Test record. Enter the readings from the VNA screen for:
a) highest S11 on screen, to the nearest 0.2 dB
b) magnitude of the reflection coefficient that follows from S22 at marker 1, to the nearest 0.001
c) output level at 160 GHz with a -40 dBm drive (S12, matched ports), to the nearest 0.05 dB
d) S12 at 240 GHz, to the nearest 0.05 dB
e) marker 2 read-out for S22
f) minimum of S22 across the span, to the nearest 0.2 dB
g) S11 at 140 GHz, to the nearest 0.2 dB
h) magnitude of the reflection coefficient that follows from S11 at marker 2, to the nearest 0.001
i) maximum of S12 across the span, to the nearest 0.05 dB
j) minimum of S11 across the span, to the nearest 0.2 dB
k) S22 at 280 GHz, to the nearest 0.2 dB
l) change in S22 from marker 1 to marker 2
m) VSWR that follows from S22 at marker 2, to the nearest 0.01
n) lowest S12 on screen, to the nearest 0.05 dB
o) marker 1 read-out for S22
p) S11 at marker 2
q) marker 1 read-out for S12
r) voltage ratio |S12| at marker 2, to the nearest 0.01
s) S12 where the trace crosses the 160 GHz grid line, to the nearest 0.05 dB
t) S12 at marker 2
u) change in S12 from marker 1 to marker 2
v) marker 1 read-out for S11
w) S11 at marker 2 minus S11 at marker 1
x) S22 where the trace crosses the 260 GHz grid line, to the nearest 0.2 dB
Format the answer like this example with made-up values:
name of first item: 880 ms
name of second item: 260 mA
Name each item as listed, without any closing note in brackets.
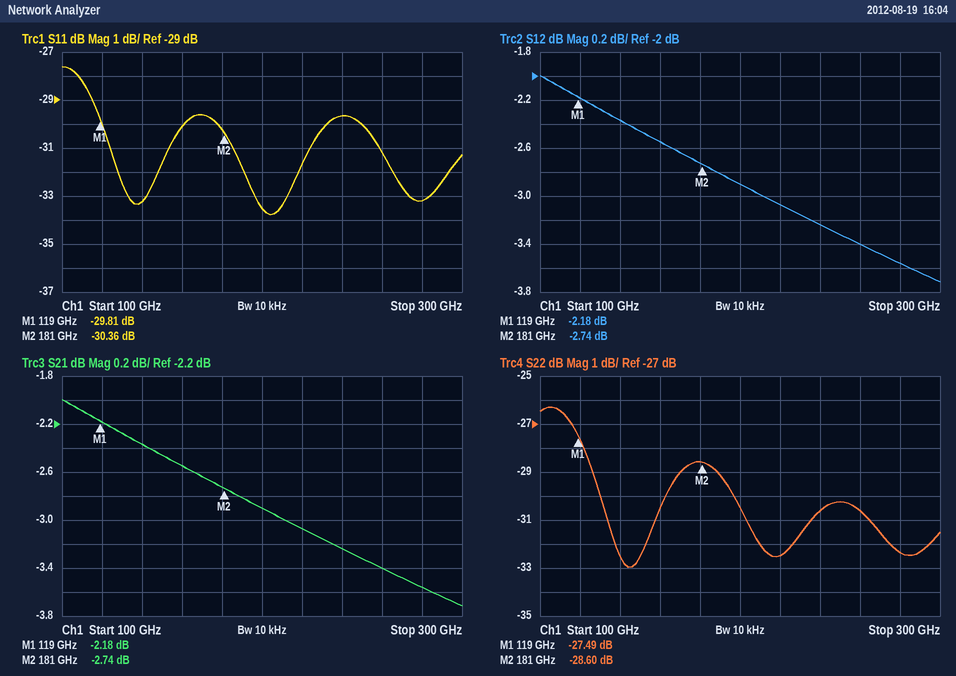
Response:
highest S11 on screen, to the nearest 0.2 dB: -27.6 dB
magnitude of the reflection coefficient that follows from S22 at marker 1, to the nearest 0.001: 0.042
output level at 160 GHz with a -40 dBm drive (S12, matched ports), to the nearest 0.05 dB: -42.55 dBm
S12 at 240 GHz, to the nearest 0.05 dB: -3.25 dB
marker 2 read-out for S22: -28.60 dB
minimum of S22 across the span, to the nearest 0.2 dB: -33.0 dB
S11 at 140 GHz, to the nearest 0.2 dB: -33.2 dB
magnitude of the reflection coefficient that follows from S11 at marker 2, to the nearest 0.001: 0.030
maximum of S12 across the span, to the nearest 0.05 dB: -2.00 dB
minimum of S11 across the span, to the nearest 0.2 dB: -33.8 dB
S22 at 280 GHz, to the nearest 0.2 dB: -32.4 dB
change in S22 from marker 1 to marker 2: -1.11 dB
VSWR that follows from S22 at marker 2, to the nearest 0.01: 1.08
lowest S12 on screen, to the nearest 0.05 dB: -3.70 dB
marker 1 read-out for S22: -27.49 dB
S11 at marker 2: -30.36 dB
marker 1 read-out for S12: -2.18 dB
voltage ratio |S12| at marker 2, to the nearest 0.01: 0.73
S12 where the trace crosses the 160 GHz grid line, to the nearest 0.05 dB: -2.55 dB
S12 at marker 2: -2.74 dB
change in S12 from marker 1 to marker 2: -0.56 dB
marker 1 read-out for S11: -29.81 dB
S11 at marker 2 minus S11 at marker 1: -0.55 dB
S22 where the trace crosses the 260 GHz grid line, to the nearest 0.2 dB: -30.6 dB
